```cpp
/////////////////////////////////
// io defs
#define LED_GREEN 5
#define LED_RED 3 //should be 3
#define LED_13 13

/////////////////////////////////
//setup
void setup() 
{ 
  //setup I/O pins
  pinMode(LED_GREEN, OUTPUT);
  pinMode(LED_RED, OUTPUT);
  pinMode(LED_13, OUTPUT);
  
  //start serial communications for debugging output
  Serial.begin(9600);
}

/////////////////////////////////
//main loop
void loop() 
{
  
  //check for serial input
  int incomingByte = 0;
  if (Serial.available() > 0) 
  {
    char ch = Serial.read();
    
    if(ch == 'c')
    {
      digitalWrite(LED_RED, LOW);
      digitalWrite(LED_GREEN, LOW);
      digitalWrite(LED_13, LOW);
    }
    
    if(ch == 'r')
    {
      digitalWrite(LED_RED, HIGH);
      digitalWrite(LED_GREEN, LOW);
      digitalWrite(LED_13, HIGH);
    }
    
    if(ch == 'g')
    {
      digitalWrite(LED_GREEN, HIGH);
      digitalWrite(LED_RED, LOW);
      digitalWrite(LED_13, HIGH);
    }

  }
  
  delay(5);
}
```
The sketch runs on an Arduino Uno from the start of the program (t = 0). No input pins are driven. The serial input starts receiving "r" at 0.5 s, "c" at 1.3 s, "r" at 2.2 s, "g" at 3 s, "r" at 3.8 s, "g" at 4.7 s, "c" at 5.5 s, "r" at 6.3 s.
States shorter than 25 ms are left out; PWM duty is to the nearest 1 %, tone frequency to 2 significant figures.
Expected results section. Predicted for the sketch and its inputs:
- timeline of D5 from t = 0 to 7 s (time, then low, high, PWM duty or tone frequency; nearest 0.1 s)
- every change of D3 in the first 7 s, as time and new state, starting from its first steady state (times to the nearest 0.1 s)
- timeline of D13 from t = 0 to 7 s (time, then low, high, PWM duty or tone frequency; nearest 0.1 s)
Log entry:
0 s low; 3 s high; 3.8 s low; 4.7 s high; 5.5 s low
0 s low; 0.5 s high; 1.3 s low; 2.2 s high; 3 s low; 3.8 s high; 4.7 s low; 6.3 s high
0 s low; 0.5 s high; 1.3 s low; 2.2 s high; 5.5 s low; 6.3 s high
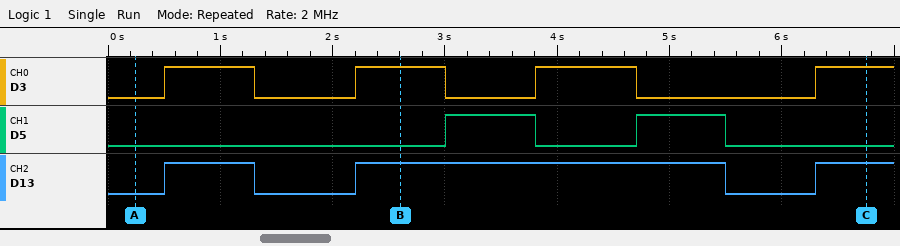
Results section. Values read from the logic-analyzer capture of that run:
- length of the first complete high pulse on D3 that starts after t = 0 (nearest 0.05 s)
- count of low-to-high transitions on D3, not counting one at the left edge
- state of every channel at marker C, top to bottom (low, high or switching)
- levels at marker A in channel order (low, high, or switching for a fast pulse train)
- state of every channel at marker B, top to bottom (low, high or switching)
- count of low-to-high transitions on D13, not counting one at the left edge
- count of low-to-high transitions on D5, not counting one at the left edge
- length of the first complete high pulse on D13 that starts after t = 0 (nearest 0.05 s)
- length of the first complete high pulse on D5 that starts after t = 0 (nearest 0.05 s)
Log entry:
0.80 s
4
D3 high, D5 low, D13 high
D3 low, D5 low, D13 low
D3 high, D5 low, D13 high
3
2
0.80 s
0.80 s
